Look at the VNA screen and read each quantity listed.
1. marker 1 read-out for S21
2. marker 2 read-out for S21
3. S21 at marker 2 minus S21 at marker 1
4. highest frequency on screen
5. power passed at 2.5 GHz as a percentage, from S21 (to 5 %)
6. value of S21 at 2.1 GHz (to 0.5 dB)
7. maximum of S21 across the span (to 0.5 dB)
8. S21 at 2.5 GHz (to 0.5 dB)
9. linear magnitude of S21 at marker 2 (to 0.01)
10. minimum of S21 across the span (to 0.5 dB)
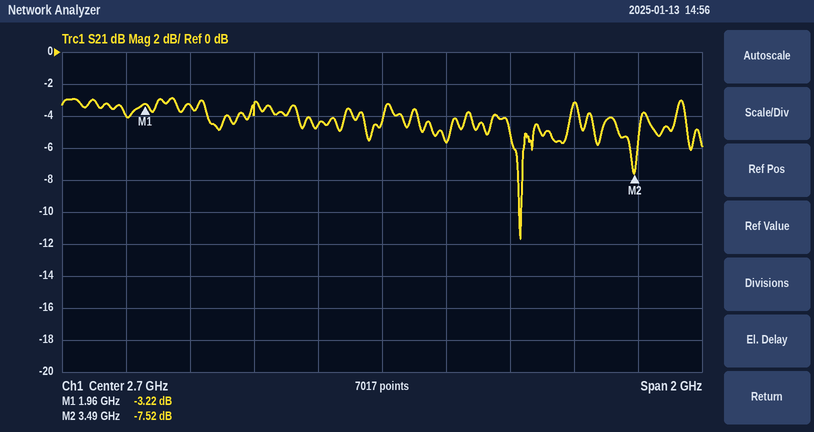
-3.22 dB
-7.52 dB
-4.30 dB
3.7 GHz
35 %
-3.5 dB
-3.0 dB
-4.5 dB
0.42
-11.5 dB
